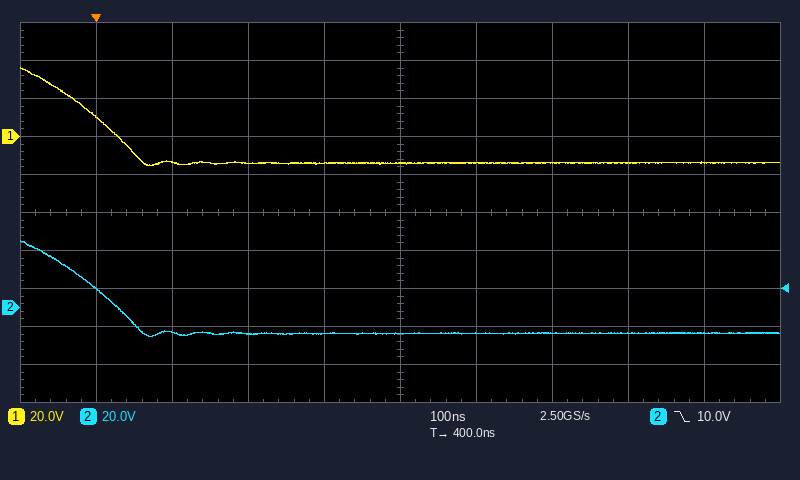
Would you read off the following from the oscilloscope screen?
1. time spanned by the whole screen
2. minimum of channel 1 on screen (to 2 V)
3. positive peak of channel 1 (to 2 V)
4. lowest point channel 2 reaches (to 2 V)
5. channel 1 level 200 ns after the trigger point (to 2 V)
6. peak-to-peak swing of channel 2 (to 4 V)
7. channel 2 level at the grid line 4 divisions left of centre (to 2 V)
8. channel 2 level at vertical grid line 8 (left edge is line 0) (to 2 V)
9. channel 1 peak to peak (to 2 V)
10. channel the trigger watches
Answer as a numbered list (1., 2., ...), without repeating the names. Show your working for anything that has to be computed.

1. 1 µs
2. -16 V
3. 36 V
4. -16 V
5. -14 V
6. 52 V
7. 10 V
8. -14 V
9. 36 V − (-16 V) = 52 V
10. channel 2
